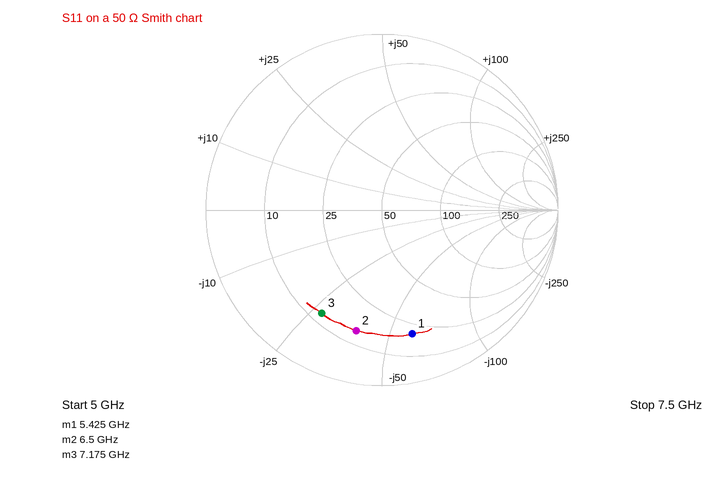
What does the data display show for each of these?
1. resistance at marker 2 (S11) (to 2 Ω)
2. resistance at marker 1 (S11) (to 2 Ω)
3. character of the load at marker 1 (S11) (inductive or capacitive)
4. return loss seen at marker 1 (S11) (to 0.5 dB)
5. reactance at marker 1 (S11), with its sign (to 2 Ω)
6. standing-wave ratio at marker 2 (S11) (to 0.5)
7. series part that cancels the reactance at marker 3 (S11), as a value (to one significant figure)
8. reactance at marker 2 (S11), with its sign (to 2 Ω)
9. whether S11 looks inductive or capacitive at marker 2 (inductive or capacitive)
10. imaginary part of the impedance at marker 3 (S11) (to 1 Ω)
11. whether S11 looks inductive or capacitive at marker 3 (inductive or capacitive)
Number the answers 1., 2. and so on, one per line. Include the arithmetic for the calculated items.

1. 14 Ω
2. 20 Ω
3. capacitive
4. 3.0 dB
5. -60 Ω
6. 5.5
7. L = 27 Ω/(2π × 7.175 GHz) ≈ 599 pH, so 600 pH to one significant figure
8. -38 Ω
9. capacitive
10. -27 Ω
11. capacitive
